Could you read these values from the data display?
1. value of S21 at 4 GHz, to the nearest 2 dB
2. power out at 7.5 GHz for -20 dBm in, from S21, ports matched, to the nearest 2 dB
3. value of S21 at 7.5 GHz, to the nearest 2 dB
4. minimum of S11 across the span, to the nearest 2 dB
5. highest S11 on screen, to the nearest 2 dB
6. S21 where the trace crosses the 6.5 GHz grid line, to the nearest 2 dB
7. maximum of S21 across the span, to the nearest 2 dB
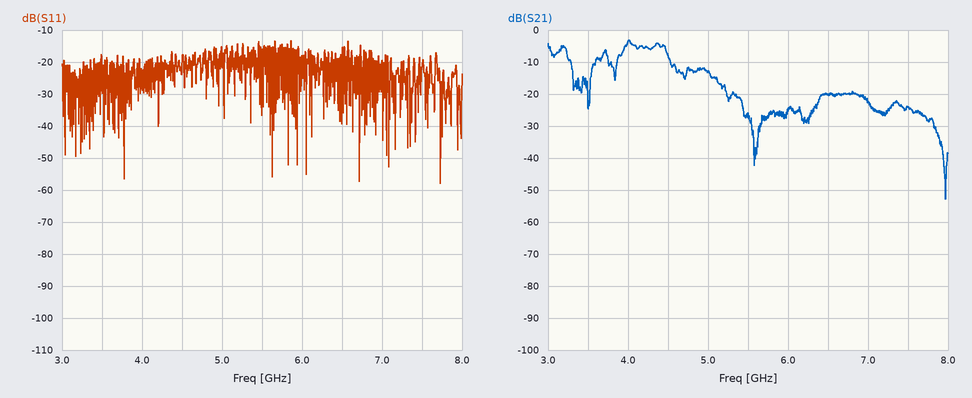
-4 dB
-44 dBm
-24 dB
-58 dB
-14 dB
-20 dB
-4 dB
